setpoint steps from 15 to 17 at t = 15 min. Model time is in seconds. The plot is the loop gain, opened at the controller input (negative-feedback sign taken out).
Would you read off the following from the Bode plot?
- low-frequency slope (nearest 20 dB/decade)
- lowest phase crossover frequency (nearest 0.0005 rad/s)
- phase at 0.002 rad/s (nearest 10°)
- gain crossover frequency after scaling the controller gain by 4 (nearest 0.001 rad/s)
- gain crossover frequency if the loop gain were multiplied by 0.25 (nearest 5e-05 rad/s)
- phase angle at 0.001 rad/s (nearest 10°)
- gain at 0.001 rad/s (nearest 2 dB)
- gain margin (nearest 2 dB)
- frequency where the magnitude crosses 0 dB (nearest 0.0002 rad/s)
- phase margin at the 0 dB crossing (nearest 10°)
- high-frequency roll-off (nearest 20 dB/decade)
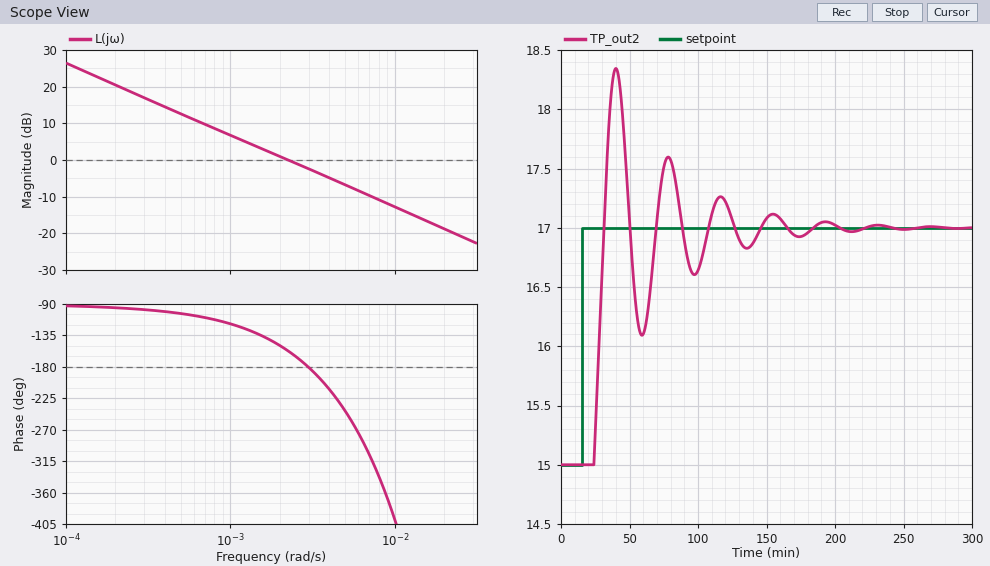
-20 dB/decade
0.0030 rad/s
-150°
0.009 rad/s
0.00055 rad/s
-120°
6 dB
2 dB
0.0022 rad/s
20°
-20 dB/decade
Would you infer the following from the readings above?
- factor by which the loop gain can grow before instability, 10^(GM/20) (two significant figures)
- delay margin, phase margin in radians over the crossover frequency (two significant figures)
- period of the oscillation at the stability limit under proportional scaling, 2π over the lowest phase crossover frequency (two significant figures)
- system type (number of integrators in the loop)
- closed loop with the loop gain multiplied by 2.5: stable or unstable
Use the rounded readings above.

1.3
160 s
2100 s
1
unstable
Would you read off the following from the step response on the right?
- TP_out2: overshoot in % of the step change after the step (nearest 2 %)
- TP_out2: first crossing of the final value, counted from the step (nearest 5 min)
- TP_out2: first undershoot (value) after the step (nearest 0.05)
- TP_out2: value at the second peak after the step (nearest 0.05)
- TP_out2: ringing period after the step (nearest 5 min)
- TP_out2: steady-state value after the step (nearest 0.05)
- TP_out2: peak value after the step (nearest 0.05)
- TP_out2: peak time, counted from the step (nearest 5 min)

68 %
15 min
16.10
17.60
40 min
17.00
18.35
25 min
